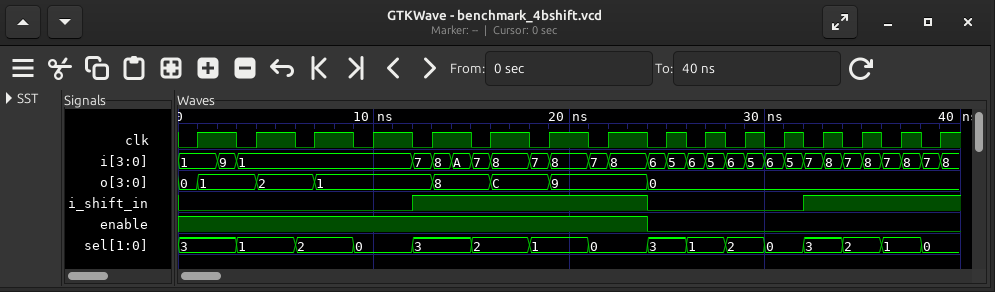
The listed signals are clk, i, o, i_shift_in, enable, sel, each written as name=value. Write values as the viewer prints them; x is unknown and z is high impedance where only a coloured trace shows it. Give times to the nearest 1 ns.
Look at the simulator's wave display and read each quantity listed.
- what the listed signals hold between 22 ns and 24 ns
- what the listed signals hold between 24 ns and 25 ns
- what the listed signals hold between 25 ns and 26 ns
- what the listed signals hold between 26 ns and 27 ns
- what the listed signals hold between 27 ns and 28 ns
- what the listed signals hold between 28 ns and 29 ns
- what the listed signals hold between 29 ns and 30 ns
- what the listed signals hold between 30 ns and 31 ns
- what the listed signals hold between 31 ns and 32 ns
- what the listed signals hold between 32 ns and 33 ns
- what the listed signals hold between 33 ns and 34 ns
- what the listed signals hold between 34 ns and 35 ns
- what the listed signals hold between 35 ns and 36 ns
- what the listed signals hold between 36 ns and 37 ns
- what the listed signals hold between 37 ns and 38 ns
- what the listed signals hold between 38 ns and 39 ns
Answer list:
clk=1, i=8, o=9, i_shift_in=1, enable=1, sel=0
clk=0, i=6, o=0, i_shift_in=0, enable=0, sel=3
clk=1, i=5, o=0, i_shift_in=0, enable=0, sel=3
clk=0, i=6, o=0, i_shift_in=0, enable=0, sel=1
clk=1, i=5, o=0, i_shift_in=0, enable=0, sel=1
clk=0, i=6, o=0, i_shift_in=0, enable=0, sel=2
clk=1, i=5, o=0, i_shift_in=0, enable=0, sel=2
clk=0, i=6, o=0, i_shift_in=0, enable=0, sel=0
clk=1, i=5, o=0, i_shift_in=0, enable=0, sel=0
clk=0, i=7, o=0, i_shift_in=1, enable=0, sel=3
clk=1, i=8, o=0, i_shift_in=1, enable=0, sel=3
clk=0, i=7, o=0, i_shift_in=1, enable=0, sel=2
clk=1, i=8, o=0, i_shift_in=1, enable=0, sel=2
clk=0, i=7, o=0, i_shift_in=1, enable=0, sel=1
clk=1, i=8, o=0, i_shift_in=1, enable=0, sel=1
clk=0, i=7, o=0, i_shift_in=1, enable=0, sel=0
